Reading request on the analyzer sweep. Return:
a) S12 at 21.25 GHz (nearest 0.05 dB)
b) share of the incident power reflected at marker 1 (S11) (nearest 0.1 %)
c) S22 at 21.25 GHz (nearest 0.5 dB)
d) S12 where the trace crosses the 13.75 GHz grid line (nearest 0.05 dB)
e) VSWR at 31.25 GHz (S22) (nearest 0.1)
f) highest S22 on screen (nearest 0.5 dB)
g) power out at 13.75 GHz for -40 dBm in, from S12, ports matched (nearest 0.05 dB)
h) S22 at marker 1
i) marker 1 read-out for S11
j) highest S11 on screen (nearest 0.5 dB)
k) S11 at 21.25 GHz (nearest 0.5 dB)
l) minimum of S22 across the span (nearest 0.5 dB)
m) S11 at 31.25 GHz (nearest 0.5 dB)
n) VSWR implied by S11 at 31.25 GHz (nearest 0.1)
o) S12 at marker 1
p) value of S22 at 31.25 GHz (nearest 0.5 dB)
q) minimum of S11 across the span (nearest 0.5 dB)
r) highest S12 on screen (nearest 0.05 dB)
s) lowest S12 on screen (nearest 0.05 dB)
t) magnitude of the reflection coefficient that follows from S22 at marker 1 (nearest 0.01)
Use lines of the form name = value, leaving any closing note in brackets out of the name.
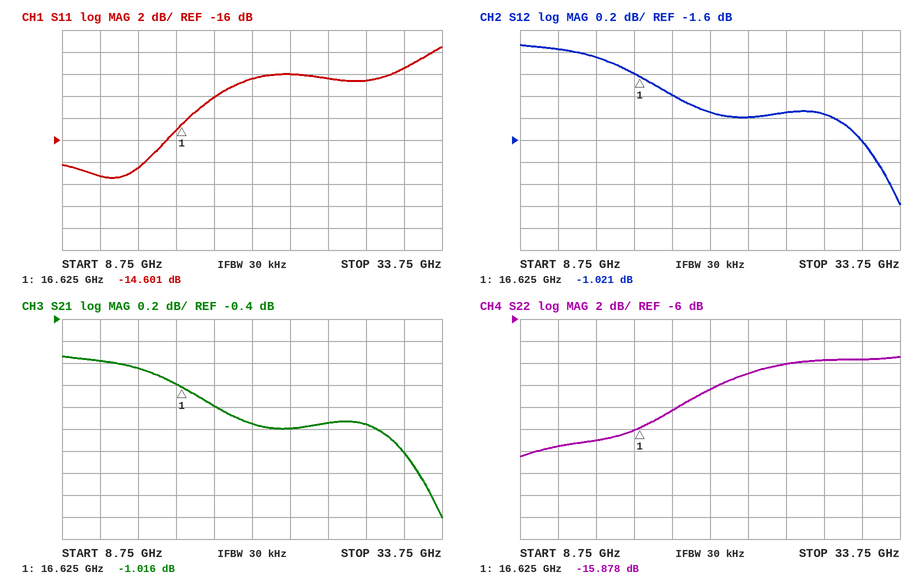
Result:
S12 at 21.25 GHz = -1.35 dB
share of the incident power reflected at marker 1 (S11) = 3.5 %
S22 at 21.25 GHz = -12.5 dB
S12 where the trace crosses the 13.75 GHz grid line = -0.85 dB
VSWR at 31.25 GHz (S22) = 2.0
highest S22 on screen = -9.5 dB
power out at 13.75 GHz for -40 dBm in, from S12, ports matched = -40.85 dBm
S22 at marker 1 = -15.878 dB
marker 1 read-out for S11 = -14.601 dB
highest S11 on screen = -7.5 dB
S11 at 21.25 GHz = -10.5 dB
minimum of S22 across the span = -18.5 dB
S11 at 31.25 GHz = -9.5 dB
VSWR implied by S11 at 31.25 GHz = 2.0
S12 at marker 1 = -1.021 dB
value of S22 at 31.25 GHz = -9.5 dB
minimum of S11 across the span = -19.5 dB
highest S12 on screen = -0.75 dB
lowest S12 on screen = -2.20 dB
magnitude of the reflection coefficient that follows from S22 at marker 1 = 0.16
